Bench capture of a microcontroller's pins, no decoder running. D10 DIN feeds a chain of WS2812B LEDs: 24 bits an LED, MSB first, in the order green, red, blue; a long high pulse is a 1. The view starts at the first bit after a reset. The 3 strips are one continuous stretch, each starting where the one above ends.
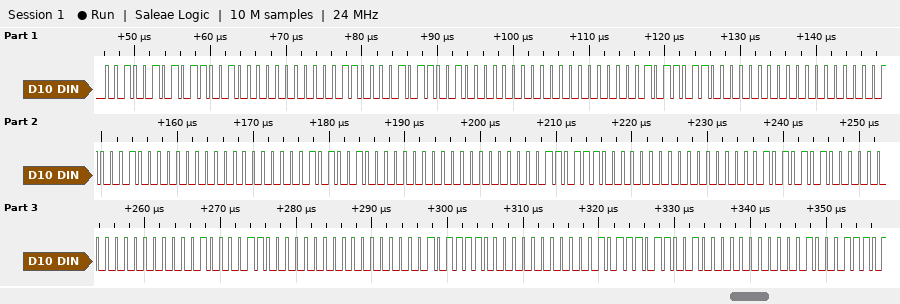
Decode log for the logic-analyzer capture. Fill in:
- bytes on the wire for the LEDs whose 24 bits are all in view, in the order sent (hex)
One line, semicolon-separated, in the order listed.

25 64 00 61 64 00 00 5B 00 00 22 00 00 52 00 00 37 00 00 55 00 00 43 00 00 5E 00 17 64 00
